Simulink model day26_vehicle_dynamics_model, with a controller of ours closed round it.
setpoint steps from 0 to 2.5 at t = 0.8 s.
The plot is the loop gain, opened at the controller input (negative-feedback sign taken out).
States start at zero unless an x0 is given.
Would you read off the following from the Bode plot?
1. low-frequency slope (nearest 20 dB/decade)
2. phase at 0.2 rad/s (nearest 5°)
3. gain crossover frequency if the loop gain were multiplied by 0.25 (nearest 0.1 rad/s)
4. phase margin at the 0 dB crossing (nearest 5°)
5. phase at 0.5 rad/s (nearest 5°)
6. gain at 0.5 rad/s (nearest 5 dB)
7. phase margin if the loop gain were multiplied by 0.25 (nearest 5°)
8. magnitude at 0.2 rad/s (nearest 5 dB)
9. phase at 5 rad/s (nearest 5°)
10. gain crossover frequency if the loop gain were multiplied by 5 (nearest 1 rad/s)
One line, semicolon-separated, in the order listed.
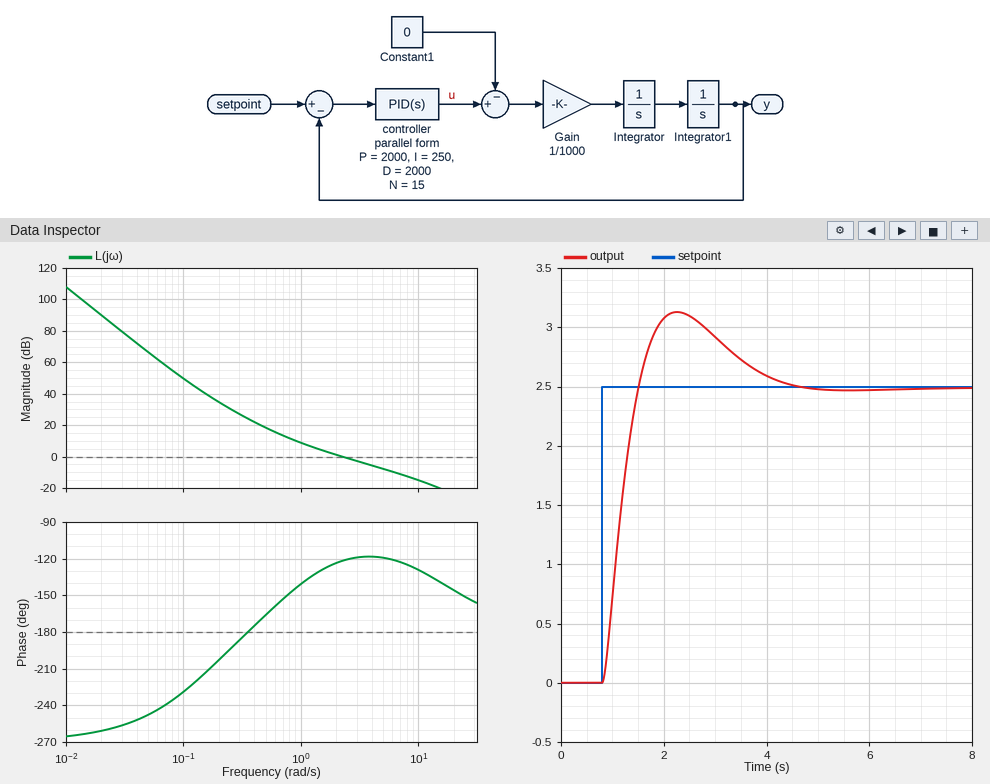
-60 dB/decade; -205°; 0.8 rad/s; 60°; -165°; 20 dB; 30°; 35 dB; -120°; 9 rad/s
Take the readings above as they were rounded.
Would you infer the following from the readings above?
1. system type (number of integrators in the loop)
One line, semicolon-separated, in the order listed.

3
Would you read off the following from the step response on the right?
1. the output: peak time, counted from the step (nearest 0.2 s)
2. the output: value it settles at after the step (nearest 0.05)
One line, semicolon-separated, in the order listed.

1.4 s; 2.50
